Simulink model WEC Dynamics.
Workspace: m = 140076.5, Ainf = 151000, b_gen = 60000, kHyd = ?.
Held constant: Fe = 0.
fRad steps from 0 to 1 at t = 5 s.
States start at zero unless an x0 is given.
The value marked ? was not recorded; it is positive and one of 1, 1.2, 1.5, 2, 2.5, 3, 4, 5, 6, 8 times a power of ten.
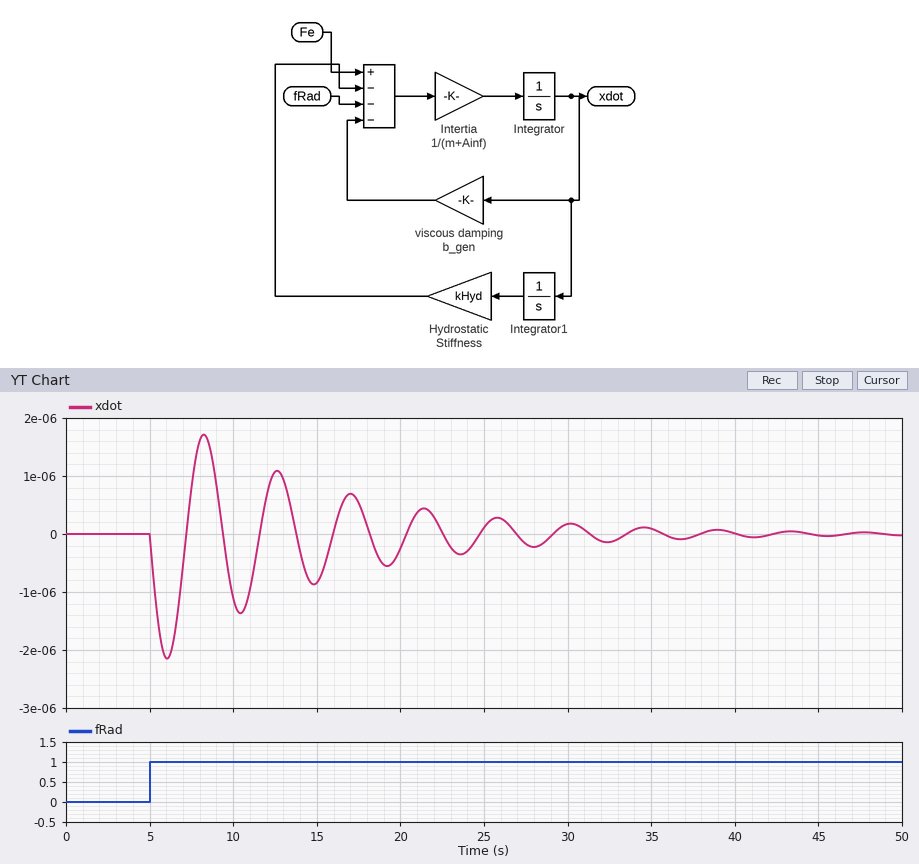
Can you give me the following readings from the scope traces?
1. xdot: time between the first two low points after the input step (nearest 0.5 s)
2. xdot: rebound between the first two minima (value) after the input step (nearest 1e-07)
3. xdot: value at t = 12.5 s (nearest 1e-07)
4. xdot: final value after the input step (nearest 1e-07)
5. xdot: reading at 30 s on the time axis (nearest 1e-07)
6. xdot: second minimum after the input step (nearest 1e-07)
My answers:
4.5 s
0.0000017
0.0000011
0.0000000
0.0000002
-0.0000014
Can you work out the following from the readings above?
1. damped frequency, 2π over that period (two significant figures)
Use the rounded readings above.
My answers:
1.4 rad/s
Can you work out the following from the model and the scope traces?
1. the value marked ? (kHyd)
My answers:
600000
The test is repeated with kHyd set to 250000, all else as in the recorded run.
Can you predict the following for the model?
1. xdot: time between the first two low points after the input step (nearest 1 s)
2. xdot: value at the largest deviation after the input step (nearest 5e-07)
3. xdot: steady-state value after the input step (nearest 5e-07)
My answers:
7 s
-0.0000030
0.0000000
